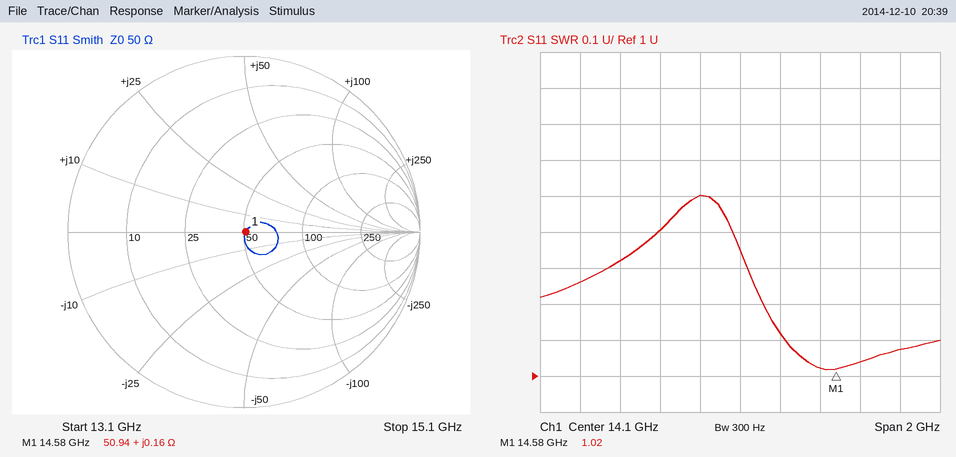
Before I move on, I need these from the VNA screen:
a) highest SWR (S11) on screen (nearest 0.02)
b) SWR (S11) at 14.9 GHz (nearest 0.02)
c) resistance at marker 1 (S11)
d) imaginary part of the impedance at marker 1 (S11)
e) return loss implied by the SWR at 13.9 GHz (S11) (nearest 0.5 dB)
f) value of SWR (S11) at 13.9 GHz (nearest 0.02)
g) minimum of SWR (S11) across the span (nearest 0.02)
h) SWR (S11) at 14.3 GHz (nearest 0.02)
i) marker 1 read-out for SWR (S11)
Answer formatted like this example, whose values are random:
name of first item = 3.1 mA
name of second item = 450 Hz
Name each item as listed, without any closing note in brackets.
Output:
highest SWR (S11) on screen = 1.50
SWR (S11) at 14.9 GHz = 1.08
resistance at marker 1 = 50.94 Ω
imaginary part of the impedance at marker 1 = +0.16 Ω
return loss implied by the SWR at 13.9 GHz (S11) = 14.0 dB
value of SWR (S11) at 13.9 GHz = 1.50
minimum of SWR (S11) across the span = 1.02
SWR (S11) at 14.3 GHz = 1.12
marker 1 read-out for SWR = 1.02
